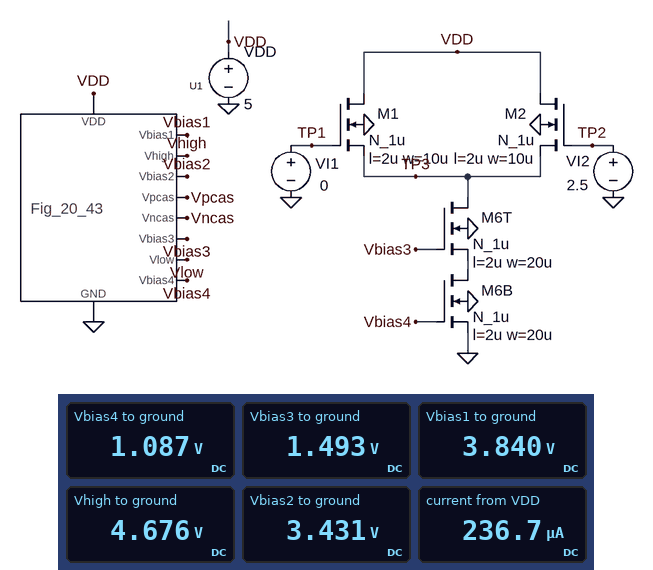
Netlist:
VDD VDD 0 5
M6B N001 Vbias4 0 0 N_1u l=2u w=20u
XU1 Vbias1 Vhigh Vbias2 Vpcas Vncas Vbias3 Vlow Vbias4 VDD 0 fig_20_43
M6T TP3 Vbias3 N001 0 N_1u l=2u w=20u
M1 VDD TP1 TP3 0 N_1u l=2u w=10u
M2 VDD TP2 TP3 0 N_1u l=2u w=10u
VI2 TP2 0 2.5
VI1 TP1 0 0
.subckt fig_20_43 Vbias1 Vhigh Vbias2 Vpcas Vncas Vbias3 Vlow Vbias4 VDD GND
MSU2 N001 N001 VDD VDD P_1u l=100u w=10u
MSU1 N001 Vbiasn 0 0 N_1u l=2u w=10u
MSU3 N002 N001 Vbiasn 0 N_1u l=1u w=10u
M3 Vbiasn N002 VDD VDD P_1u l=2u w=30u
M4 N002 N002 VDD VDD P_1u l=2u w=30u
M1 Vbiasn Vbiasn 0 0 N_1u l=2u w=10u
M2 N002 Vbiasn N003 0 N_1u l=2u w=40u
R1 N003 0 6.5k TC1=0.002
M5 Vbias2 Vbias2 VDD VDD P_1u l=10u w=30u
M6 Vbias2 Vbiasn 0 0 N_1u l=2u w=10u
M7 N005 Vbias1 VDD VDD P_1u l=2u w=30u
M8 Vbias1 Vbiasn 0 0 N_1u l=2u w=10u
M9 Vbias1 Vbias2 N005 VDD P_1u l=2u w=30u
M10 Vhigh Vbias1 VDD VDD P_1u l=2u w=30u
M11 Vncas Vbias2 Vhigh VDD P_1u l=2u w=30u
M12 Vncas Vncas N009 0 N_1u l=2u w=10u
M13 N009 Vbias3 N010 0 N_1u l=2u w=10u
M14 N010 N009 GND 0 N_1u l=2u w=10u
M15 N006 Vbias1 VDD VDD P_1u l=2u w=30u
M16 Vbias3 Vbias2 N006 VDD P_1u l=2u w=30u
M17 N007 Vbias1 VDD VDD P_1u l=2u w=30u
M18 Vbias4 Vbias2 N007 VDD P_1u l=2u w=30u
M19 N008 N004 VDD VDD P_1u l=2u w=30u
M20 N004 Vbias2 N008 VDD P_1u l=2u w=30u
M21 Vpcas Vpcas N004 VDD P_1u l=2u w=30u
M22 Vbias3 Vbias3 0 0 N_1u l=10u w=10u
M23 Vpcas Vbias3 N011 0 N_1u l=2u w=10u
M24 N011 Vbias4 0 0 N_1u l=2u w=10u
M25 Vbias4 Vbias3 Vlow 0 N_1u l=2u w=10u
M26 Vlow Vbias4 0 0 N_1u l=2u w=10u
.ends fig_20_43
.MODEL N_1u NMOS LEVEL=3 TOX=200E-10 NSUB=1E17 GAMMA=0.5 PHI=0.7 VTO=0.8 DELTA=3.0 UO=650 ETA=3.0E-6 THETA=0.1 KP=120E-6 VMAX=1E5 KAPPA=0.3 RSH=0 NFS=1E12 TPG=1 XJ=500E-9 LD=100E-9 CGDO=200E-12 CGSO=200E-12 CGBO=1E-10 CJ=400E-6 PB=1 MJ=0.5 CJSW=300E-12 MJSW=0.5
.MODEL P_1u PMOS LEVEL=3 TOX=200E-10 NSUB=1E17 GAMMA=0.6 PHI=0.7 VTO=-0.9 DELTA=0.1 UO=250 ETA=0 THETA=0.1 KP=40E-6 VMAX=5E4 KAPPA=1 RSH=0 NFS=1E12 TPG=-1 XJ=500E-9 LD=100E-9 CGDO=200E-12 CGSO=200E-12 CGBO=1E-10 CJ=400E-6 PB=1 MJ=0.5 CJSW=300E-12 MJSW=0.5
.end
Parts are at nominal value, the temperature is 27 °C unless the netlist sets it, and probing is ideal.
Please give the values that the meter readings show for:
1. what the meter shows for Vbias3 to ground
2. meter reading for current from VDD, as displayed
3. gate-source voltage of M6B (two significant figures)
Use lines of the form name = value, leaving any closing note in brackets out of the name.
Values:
what the meter shows for Vbias3 to ground = 1.493 V
meter reading for current from VDD, as displayed = 236.7 µA
gate-source voltage of M6B = 1.1 V
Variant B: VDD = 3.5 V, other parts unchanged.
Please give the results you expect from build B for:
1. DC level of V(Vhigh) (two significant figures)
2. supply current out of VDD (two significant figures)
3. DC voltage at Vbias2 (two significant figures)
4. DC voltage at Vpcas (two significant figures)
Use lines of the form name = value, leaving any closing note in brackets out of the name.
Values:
DC level of V(Vhigh) = 3.2 V
supply current out of VDD = 210 µA
DC voltage at Vbias2 = 2.0 V
DC voltage at Vpcas = 940 mV
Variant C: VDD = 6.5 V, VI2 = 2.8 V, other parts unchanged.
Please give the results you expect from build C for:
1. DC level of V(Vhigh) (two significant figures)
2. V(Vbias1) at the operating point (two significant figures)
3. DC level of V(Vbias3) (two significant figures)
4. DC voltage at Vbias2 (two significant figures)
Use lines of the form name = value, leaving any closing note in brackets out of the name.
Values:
DC level of V(Vhigh) = 6.2 V
V(Vbias1) at the operating point = 5.3 V
DC level of V(Vbias3) = 1.5 V
DC voltage at Vbias2 = 4.9 V
